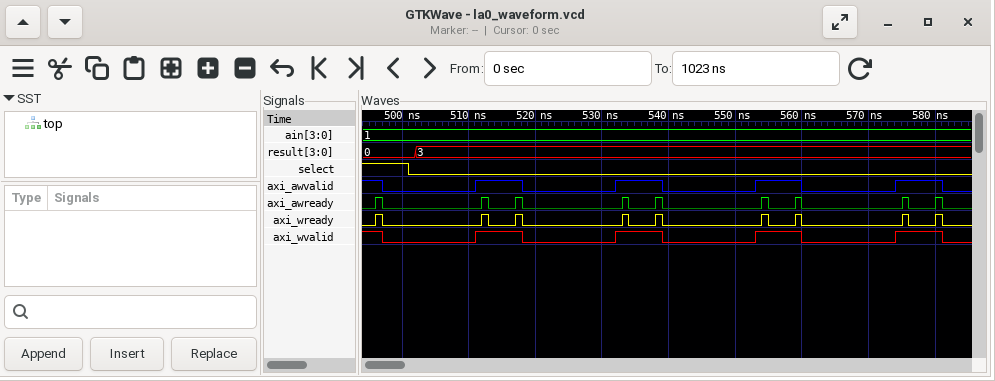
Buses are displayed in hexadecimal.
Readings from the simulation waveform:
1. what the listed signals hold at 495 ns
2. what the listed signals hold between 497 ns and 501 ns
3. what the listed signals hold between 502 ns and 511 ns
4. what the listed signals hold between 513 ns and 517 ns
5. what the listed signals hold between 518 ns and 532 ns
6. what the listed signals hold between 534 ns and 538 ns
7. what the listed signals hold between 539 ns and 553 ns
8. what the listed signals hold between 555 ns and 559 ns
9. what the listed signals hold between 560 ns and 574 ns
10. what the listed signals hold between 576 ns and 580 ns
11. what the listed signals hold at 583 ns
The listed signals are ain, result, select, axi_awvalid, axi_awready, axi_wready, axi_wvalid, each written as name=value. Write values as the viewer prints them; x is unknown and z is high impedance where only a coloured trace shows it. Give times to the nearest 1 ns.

ain=1, result=0, select=1, axi_awvalid=1, axi_awready=0, axi_wready=0, axi_wvalid=1
ain=1, result=0, select=1, axi_awvalid=0, axi_awready=0, axi_wready=0, axi_wvalid=0
ain=1, result=3, select=0, axi_awvalid=0, axi_awready=0, axi_wready=0, axi_wvalid=0
ain=1, result=3, select=0, axi_awvalid=1, axi_awready=0, axi_wready=0, axi_wvalid=1
ain=1, result=3, select=0, axi_awvalid=0, axi_awready=0, axi_wready=0, axi_wvalid=0
ain=1, result=3, select=0, axi_awvalid=1, axi_awready=0, axi_wready=0, axi_wvalid=1
ain=1, result=3, select=0, axi_awvalid=0, axi_awready=0, axi_wready=0, axi_wvalid=0
ain=1, result=3, select=0, axi_awvalid=1, axi_awready=0, axi_wready=0, axi_wvalid=1
ain=1, result=3, select=0, axi_awvalid=0, axi_awready=0, axi_wready=0, axi_wvalid=0
ain=1, result=3, select=0, axi_awvalid=1, axi_awready=0, axi_wready=0, axi_wvalid=1
ain=1, result=3, select=0, axi_awvalid=0, axi_awready=0, axi_wready=0, axi_wvalid=0
